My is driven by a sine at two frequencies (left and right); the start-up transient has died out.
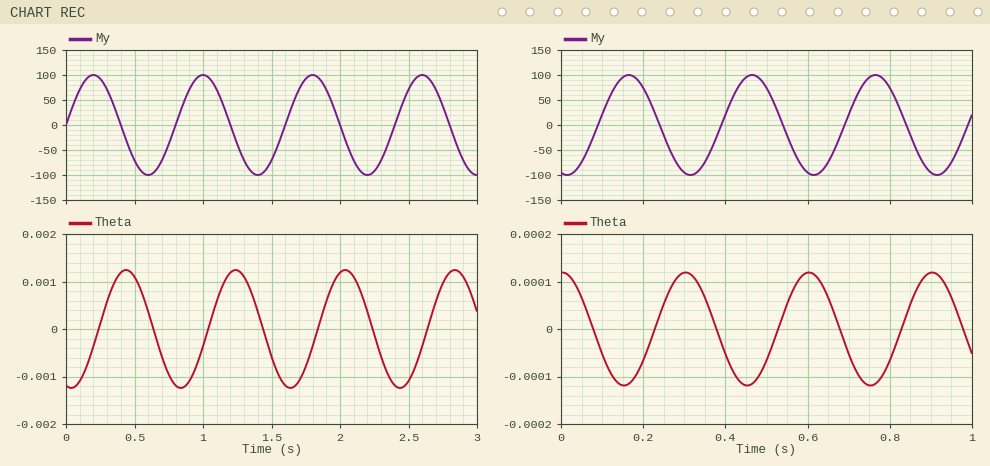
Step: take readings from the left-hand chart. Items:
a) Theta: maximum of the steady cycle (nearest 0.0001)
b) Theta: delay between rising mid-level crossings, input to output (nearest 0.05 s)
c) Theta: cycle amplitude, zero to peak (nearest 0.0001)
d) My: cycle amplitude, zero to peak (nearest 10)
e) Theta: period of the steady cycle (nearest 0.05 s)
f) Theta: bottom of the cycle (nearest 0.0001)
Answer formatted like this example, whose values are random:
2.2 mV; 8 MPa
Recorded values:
0.0012; 0.25 s; 0.0012; 100; 0.80 s; -0.0012
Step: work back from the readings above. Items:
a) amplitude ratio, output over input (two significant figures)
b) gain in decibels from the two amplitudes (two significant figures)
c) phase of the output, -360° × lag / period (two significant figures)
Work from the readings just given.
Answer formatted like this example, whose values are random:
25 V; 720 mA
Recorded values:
0.000012; -98 dB; -110°
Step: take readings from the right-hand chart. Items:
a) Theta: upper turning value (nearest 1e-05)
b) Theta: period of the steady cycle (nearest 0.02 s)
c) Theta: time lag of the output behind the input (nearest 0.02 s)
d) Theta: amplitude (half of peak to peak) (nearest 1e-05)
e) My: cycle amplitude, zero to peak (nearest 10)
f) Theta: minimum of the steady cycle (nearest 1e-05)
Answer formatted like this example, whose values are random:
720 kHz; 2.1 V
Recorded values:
0.00012; 0.30 s; 0.14 s; 0.00012; 100; -0.00012
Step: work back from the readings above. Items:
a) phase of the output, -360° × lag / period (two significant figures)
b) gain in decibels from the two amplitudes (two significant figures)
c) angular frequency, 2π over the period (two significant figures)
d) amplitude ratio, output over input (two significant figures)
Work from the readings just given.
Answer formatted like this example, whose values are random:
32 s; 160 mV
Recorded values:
-170°; -120 dB; 21 rad/s; 0.0000012
